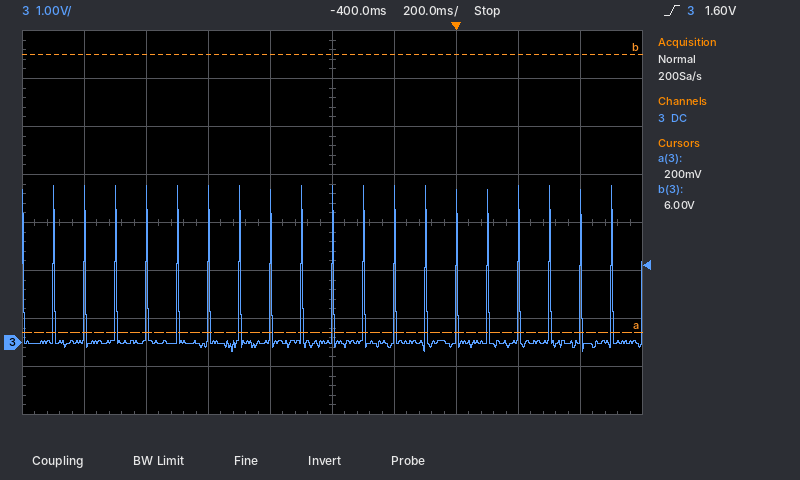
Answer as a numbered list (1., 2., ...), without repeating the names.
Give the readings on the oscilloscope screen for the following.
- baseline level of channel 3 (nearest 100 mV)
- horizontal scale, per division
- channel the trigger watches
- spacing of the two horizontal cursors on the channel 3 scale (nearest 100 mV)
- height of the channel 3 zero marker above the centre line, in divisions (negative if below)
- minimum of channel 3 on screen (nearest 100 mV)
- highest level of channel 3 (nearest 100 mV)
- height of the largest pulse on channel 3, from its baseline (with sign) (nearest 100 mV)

1. 0.0 V
2. 200 ms
3. channel 3
4. 5.8 V
5. -2.5 div
6. -200 mV
7. 3.3 V
8. +3.3 V
